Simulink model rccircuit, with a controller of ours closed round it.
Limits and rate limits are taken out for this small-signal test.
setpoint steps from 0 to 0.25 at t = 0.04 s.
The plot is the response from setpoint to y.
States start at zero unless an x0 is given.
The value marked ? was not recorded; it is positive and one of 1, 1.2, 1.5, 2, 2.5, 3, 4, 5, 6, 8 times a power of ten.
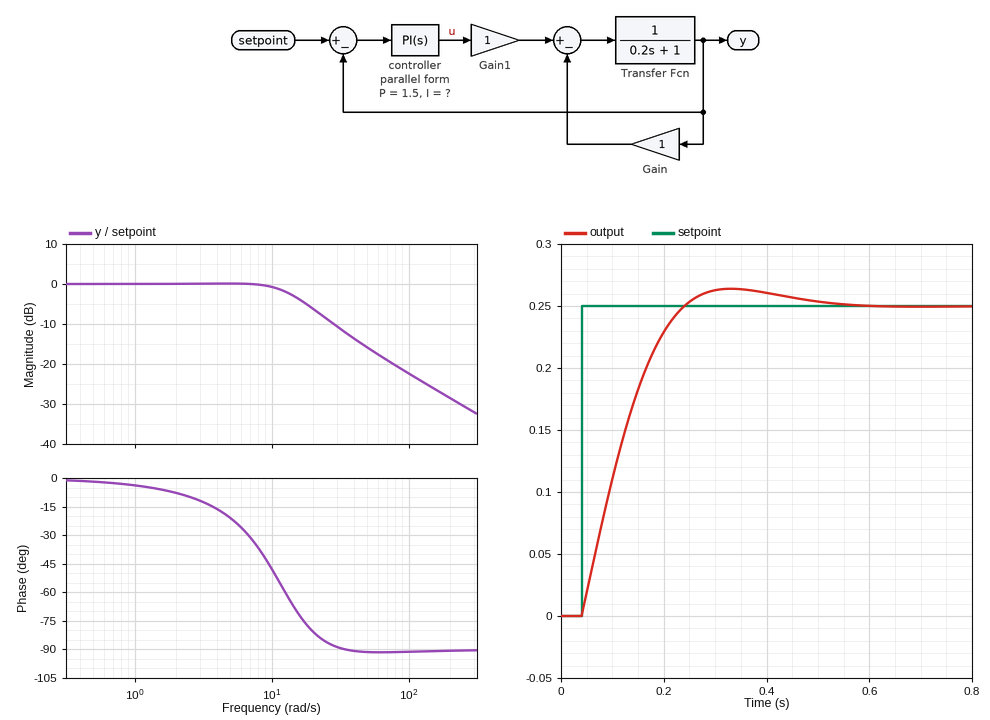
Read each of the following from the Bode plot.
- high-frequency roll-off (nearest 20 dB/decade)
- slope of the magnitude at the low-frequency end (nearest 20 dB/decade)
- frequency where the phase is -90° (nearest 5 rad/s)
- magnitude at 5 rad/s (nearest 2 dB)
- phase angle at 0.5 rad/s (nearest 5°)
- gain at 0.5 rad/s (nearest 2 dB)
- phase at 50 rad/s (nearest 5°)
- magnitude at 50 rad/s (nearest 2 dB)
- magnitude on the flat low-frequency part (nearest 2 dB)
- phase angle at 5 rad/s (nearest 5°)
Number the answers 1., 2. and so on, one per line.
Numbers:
1. -20 dB/decade
2. 0 dB/decade
3. 35 rad/s
4. 0 dB
5. 0°
6. 0 dB
7. -90°
8. -16 dB
9. 0 dB
10. -20°
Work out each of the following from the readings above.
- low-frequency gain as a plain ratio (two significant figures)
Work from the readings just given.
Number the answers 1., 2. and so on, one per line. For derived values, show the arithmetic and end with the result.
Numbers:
1. 10^(0 / 20) = 1.0
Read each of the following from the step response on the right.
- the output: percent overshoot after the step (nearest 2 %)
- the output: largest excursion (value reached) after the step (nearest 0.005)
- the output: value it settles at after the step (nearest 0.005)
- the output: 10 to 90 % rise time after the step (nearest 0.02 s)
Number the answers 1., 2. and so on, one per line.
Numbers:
1. 6 %
2. 0.265
3. 0.250
4. 0.14 s
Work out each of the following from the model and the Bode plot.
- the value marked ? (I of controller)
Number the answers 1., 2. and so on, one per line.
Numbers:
1. 30
